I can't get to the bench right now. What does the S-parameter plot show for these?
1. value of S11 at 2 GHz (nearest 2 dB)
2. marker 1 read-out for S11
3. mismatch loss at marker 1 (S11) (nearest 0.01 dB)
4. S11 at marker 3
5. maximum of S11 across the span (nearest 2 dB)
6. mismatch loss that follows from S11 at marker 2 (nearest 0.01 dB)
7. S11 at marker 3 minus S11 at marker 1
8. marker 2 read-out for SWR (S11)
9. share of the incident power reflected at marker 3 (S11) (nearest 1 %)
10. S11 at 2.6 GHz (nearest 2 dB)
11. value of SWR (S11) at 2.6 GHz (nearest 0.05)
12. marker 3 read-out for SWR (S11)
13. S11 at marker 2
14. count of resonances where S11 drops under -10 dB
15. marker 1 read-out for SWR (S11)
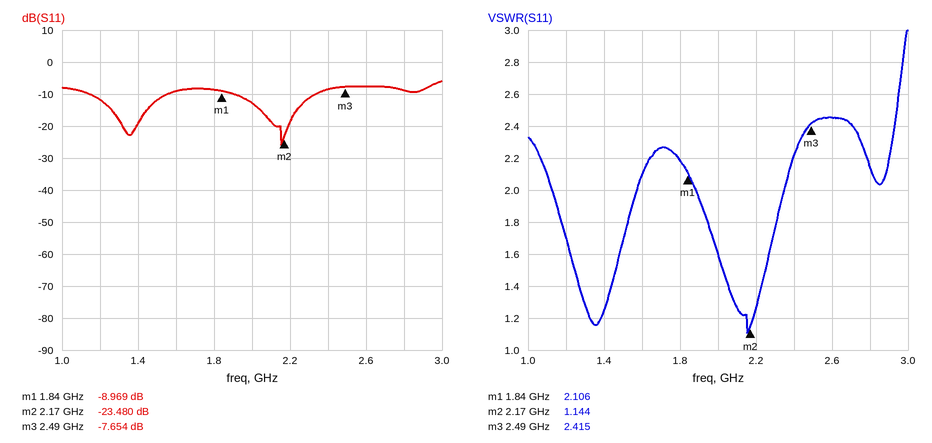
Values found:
-12 dB
-8.969 dB
0.59 dB
-7.654 dB
-6 dB
0.02 dB
1.315 dB
1.144
17 %
-8 dB
2.45
2.415
-23.480 dB
2
2.106
